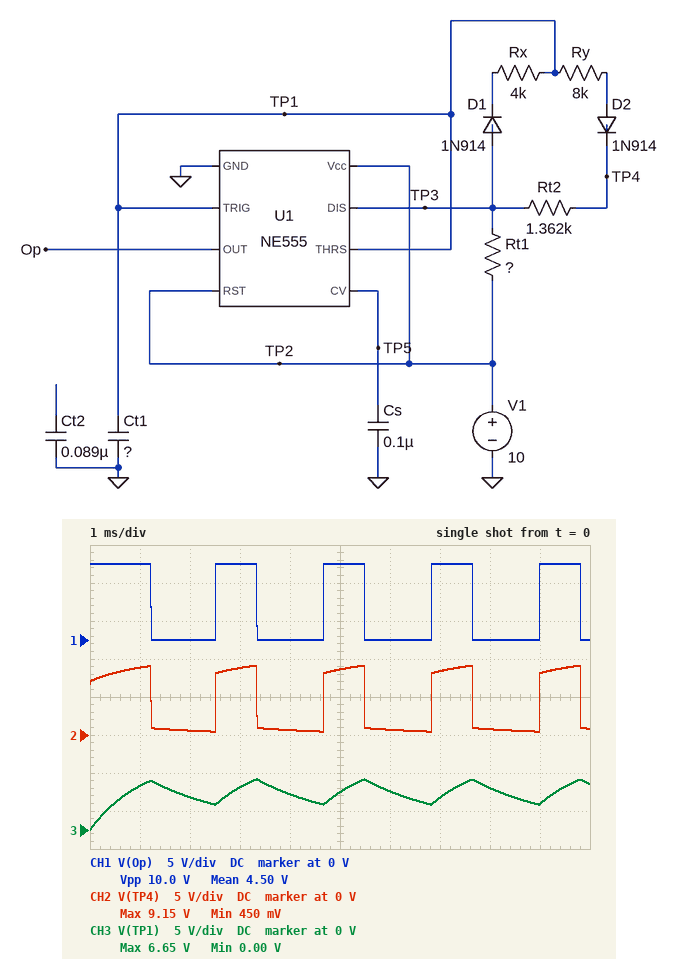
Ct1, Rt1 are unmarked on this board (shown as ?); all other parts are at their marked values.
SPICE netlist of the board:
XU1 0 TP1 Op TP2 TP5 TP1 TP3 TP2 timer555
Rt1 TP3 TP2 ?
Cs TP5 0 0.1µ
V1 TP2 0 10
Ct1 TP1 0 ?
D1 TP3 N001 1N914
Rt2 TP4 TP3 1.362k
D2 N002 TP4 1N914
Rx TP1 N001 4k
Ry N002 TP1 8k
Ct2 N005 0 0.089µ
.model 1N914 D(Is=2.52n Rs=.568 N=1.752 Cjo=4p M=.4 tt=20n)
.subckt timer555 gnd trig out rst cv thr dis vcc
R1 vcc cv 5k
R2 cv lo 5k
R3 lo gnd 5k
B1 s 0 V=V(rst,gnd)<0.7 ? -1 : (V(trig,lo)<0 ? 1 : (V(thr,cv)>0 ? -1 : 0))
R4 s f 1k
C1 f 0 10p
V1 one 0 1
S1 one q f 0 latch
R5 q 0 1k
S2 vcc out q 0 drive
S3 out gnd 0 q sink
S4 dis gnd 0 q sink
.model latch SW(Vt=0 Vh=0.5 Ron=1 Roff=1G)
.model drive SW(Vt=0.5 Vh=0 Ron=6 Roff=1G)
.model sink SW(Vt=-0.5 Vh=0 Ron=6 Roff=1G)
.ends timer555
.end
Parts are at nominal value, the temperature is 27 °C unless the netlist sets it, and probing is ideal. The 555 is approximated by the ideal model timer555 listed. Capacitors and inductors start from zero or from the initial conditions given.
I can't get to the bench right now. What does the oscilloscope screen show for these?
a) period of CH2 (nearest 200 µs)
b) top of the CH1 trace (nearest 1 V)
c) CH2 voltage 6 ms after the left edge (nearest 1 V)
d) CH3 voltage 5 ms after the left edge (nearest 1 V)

2.2 ms
10 V
1 V
5 V
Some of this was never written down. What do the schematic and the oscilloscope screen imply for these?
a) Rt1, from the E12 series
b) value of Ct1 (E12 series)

1.8 kΩ
180 nF
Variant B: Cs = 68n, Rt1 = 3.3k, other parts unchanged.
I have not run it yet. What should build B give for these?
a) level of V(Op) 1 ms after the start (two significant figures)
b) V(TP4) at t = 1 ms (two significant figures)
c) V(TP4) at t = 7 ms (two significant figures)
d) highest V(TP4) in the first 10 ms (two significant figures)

10 V
8.0 V
620 mV
8.7 V
